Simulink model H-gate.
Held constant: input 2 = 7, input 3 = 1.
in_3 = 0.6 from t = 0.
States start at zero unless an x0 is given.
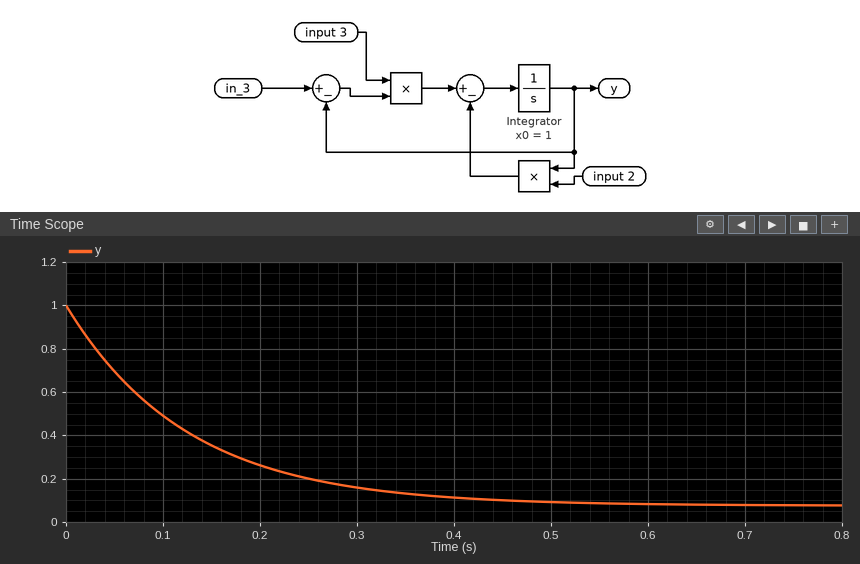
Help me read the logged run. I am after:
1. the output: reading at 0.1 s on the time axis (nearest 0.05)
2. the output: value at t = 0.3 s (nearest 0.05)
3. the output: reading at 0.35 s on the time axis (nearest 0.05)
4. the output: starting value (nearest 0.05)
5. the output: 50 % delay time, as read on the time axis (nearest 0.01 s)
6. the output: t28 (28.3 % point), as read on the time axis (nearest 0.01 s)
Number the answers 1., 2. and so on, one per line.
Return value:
1. 0.50
2. 0.15
3. 0.15
4. 1.00
5. 0.09 s
6. 0.04 s
